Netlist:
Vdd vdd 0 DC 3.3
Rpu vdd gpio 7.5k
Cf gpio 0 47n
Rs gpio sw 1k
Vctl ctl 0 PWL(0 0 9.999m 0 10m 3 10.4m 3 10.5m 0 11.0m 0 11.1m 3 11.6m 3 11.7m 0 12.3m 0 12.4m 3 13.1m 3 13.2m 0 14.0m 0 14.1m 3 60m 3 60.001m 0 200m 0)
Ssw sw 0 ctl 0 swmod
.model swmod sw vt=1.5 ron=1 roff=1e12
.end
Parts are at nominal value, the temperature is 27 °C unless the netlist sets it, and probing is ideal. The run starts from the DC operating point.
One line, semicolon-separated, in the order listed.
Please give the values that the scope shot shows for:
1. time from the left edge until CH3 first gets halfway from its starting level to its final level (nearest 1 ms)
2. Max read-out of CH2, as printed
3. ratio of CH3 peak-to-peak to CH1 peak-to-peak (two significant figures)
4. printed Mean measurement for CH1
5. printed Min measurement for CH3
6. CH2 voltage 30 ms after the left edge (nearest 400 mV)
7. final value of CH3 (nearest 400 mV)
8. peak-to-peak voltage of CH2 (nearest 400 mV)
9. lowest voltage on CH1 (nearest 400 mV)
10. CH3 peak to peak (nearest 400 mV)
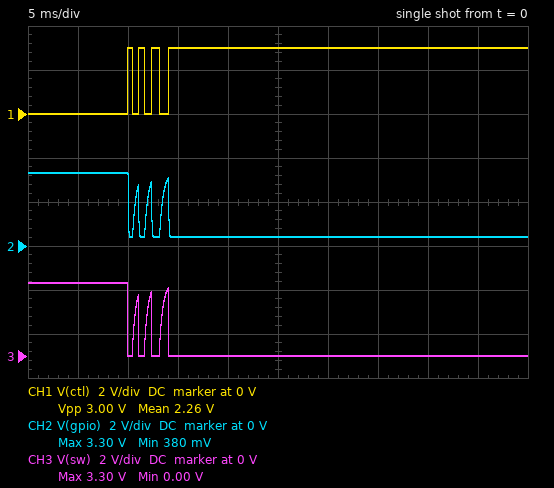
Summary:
10 ms; 3.30 V; 1.1; 2.26 V; 0.00 V; 400 mV; 0 V; 2.8 V; 0 V; 3.2 V
